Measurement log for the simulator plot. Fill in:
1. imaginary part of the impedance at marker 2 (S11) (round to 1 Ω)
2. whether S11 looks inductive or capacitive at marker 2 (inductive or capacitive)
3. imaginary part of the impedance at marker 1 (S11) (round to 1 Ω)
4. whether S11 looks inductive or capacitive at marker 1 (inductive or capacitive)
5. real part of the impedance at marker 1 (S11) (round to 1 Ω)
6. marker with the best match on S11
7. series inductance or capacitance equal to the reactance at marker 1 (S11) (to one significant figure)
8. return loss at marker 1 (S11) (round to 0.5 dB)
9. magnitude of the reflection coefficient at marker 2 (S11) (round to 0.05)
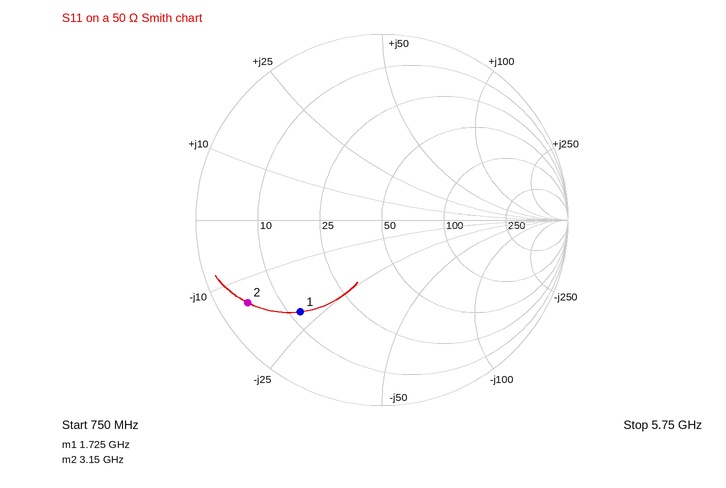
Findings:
-14 Ω
capacitive
-21 Ω
capacitive
12 Ω
marker 1
4 pF
3.5 dB
0.85
